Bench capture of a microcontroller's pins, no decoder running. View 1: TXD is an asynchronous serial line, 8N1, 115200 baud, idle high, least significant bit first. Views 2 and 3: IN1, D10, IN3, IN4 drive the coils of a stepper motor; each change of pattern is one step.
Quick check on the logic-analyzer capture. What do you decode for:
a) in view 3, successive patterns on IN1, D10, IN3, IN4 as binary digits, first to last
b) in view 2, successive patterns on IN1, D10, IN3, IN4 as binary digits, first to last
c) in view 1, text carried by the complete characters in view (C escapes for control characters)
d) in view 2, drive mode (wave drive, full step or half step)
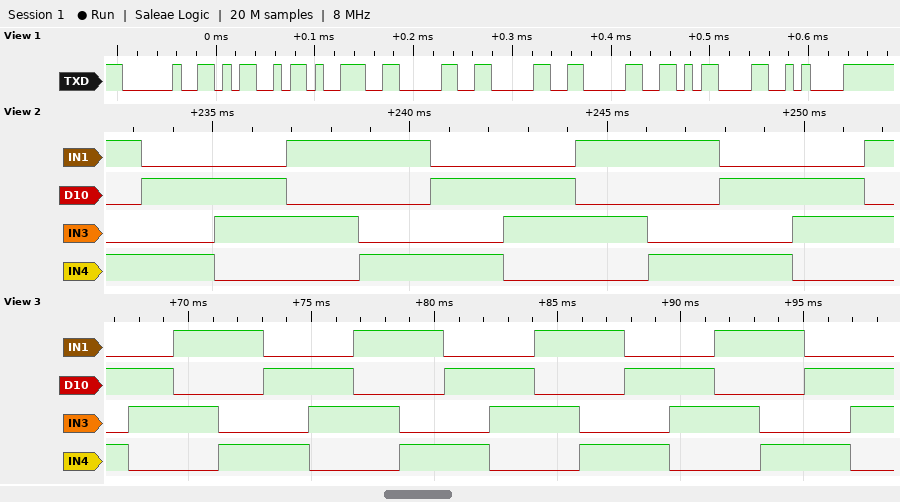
0101 0110 1010 1001 0101 0110 1010 1001 0101 0110 1010 1001 0101 0110 1010 1001 0101 0110
1001 0101 0110 1010 1001 0101 0110 1010 1001 0101 0110 1010
" M9000\r\n"
full step
